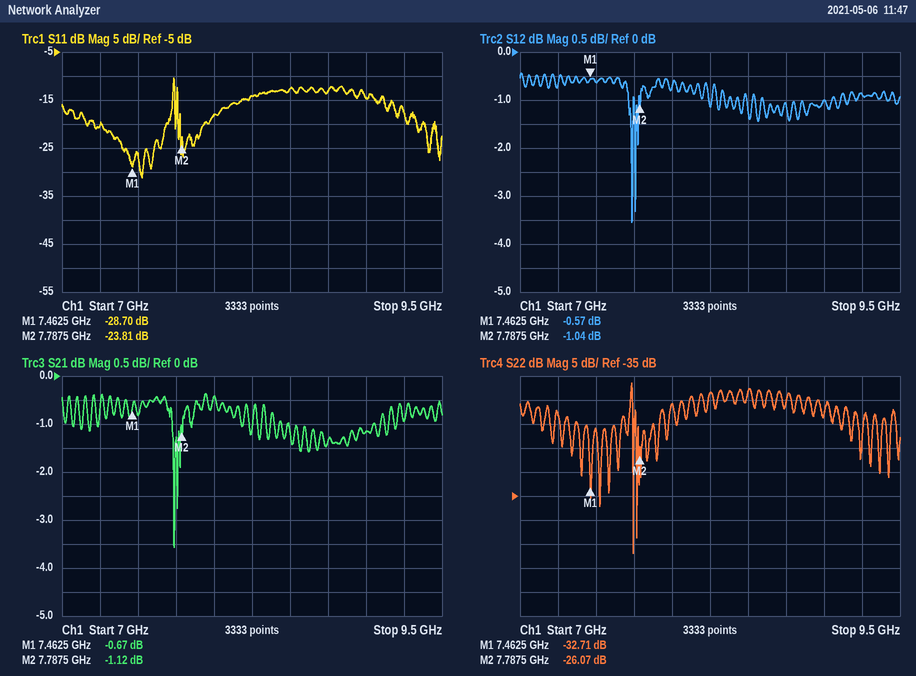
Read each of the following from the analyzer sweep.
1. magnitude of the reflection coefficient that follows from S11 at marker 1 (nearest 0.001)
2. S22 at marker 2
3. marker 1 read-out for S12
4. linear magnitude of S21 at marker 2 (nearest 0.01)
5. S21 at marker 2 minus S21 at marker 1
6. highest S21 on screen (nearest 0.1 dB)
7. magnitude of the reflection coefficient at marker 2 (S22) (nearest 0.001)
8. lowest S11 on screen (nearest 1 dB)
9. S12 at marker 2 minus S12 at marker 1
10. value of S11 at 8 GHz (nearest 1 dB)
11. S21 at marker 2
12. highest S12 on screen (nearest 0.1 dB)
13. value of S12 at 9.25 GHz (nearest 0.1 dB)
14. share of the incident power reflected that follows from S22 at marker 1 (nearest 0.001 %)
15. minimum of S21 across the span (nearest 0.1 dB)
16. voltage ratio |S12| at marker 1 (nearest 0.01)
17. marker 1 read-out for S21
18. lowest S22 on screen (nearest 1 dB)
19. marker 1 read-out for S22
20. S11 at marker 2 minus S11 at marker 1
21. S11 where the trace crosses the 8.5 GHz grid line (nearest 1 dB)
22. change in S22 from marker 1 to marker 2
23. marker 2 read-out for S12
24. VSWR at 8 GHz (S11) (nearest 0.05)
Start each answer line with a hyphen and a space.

- 0.037
- -26.07 dB
- -0.57 dB
- 0.88
- -0.45 dB
- -0.4 dB
- 0.050
- -31 dB
- -0.47 dB
- -18 dB
- -1.12 dB
- -0.4 dB
- -0.9 dB
- 0.054 %
- -3.6 dB
- 0.94
- -0.67 dB
- -47 dB
- -32.71 dB
- 4.89 dB
- -13 dB
- 6.64 dB
- -1.04 dB
- 1.30
